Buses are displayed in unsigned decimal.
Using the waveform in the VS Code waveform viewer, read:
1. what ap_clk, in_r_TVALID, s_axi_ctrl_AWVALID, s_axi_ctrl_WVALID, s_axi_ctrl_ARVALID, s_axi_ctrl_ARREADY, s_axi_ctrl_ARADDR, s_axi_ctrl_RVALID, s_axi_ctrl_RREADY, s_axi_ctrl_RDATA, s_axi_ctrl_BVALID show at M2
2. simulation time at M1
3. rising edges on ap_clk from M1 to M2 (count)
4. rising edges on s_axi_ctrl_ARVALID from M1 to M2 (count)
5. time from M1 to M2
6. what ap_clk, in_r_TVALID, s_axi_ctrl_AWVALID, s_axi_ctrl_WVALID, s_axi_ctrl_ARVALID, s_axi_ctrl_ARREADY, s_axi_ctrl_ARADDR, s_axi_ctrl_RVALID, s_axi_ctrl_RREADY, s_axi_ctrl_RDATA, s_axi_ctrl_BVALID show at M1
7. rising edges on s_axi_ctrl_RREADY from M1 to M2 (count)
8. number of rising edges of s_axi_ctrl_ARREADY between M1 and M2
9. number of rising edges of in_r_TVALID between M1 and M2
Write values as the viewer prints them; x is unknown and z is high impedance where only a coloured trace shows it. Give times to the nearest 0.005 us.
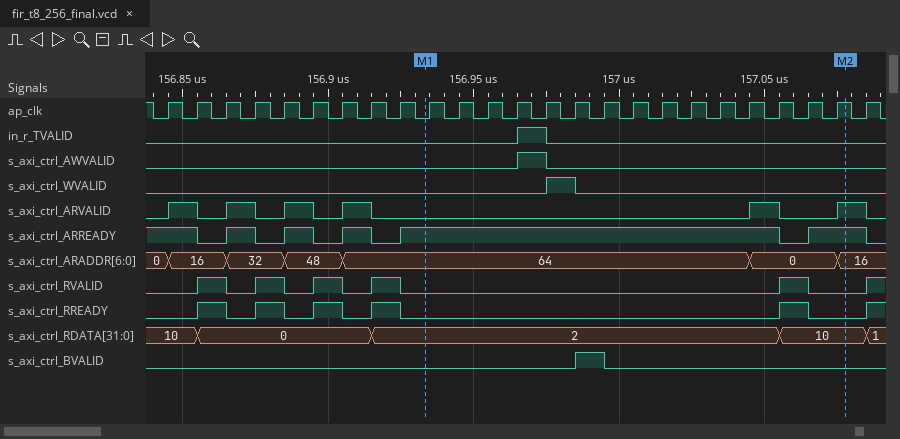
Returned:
ap_clk=1, in_r_TVALID=0, s_axi_ctrl_AWVALID=0, s_axi_ctrl_WVALID=0, s_axi_ctrl_ARVALID=1, s_axi_ctrl_ARREADY=1, s_axi_ctrl_ARADDR=16, s_axi_ctrl_RVALID=0, s_axi_ctrl_RREADY=0, s_axi_ctrl_RDATA=10, s_axi_ctrl_BVALID=0
156.935 us
15
2
0.145 us
ap_clk=0, in_r_TVALID=0, s_axi_ctrl_AWVALID=0, s_axi_ctrl_WVALID=0, s_axi_ctrl_ARVALID=0, s_axi_ctrl_ARREADY=1, s_axi_ctrl_ARADDR=64, s_axi_ctrl_RVALID=0, s_axi_ctrl_RREADY=0, s_axi_ctrl_RDATA=2, s_axi_ctrl_BVALID=0
1
1
1
